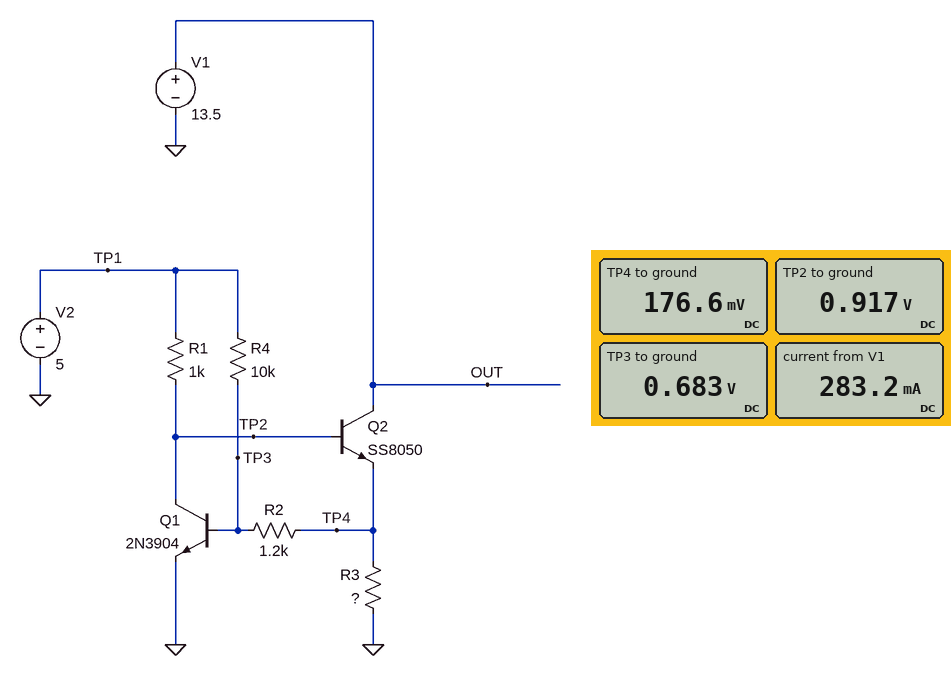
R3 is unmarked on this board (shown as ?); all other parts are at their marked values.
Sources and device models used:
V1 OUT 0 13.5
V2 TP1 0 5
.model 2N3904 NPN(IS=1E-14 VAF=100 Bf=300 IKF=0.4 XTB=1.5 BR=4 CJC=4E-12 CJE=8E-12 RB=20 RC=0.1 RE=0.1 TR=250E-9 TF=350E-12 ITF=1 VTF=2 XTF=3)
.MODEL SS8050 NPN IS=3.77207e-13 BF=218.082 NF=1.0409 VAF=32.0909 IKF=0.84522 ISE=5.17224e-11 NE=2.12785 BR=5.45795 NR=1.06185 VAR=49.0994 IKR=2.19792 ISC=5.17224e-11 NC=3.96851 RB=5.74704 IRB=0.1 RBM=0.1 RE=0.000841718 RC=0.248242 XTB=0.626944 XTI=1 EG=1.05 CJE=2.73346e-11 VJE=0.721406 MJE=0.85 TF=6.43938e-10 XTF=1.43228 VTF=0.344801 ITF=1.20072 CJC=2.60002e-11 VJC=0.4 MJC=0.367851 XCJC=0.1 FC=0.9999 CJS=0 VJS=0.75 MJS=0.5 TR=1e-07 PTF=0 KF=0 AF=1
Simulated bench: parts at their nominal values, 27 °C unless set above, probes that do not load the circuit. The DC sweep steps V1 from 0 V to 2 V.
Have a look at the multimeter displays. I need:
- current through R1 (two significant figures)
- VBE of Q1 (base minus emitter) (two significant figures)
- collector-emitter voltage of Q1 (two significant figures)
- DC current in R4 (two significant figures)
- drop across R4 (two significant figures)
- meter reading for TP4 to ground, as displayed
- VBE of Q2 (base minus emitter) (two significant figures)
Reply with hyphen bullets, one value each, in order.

- 4.1 mA
- 680 mV
- 920 mV
- 430 µA
- 4.3 V
- 176.6 mV
- 740 mV
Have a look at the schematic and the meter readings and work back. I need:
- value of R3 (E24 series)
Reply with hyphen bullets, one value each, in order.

- 0.62 Ω
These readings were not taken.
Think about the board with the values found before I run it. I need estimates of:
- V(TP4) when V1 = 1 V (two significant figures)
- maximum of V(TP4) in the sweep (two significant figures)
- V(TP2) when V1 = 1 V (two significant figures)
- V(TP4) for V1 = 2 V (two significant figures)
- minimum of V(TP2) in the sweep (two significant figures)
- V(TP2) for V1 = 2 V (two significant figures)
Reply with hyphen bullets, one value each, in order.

- 170 mV
- 170 mV
- 920 mV
- 170 mV
- 700 mV
- 920 mV
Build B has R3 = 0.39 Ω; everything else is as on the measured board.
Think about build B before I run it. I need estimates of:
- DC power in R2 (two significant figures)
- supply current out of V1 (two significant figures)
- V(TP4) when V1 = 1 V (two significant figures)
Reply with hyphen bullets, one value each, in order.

- 220 µW
- 420 mA
- 150 mV
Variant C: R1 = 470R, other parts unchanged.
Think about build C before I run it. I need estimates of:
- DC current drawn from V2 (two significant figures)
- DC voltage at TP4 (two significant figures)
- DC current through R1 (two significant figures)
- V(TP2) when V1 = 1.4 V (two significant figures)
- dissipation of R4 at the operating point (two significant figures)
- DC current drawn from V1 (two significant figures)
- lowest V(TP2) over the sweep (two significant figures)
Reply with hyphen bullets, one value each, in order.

- 9.0 mA
- 220 mV
- 8.6 mA
- 980 mV
- 1.8 mW
- 350 mA
- 750 mV
